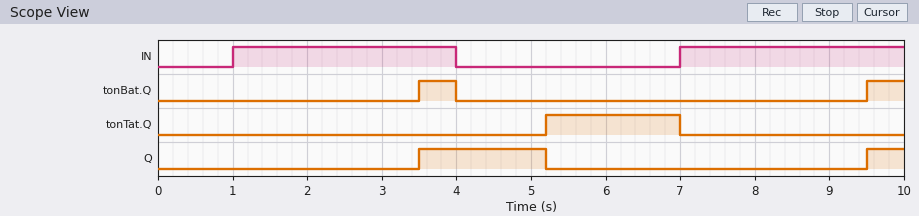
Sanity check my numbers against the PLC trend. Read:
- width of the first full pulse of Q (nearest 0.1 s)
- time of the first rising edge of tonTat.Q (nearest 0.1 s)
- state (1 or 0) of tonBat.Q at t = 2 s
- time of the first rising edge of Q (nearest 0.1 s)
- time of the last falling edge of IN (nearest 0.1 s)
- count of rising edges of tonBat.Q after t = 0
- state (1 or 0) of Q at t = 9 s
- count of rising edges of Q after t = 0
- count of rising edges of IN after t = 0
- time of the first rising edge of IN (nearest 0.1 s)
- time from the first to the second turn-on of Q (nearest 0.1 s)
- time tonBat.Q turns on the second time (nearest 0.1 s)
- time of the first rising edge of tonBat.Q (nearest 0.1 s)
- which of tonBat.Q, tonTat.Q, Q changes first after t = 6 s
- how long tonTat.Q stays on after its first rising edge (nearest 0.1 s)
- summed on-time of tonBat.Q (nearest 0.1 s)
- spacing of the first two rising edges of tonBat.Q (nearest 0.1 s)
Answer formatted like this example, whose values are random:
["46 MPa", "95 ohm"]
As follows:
["1.7 s", "5.2 s", "0", "3.5 s", "4.0 s", "2", "0", "2", "2", "1.0 s", "6.0 s", "9.5 s", "3.5 s", "tonTat.Q", "1.8 s", "1.0 s", "6.0 s"]
